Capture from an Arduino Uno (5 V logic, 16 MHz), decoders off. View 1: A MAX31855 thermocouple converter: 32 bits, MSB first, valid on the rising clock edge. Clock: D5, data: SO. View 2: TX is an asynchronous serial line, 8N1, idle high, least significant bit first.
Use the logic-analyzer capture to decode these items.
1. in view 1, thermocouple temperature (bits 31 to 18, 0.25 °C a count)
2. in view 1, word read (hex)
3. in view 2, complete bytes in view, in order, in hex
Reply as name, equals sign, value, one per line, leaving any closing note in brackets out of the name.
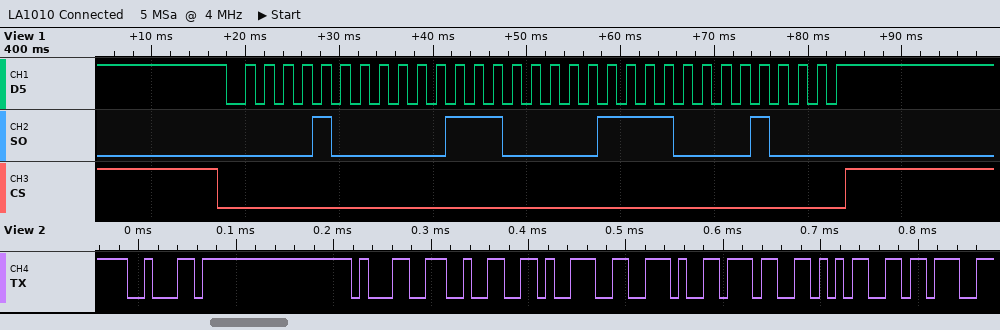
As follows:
in view 1, thermocouple temperature = 129.75 °C
in view 1, word read = 0x081C1E10
in view 2, complete bytes in view, in order, in hex = 62 31 32 39 2E 37 35 3B
